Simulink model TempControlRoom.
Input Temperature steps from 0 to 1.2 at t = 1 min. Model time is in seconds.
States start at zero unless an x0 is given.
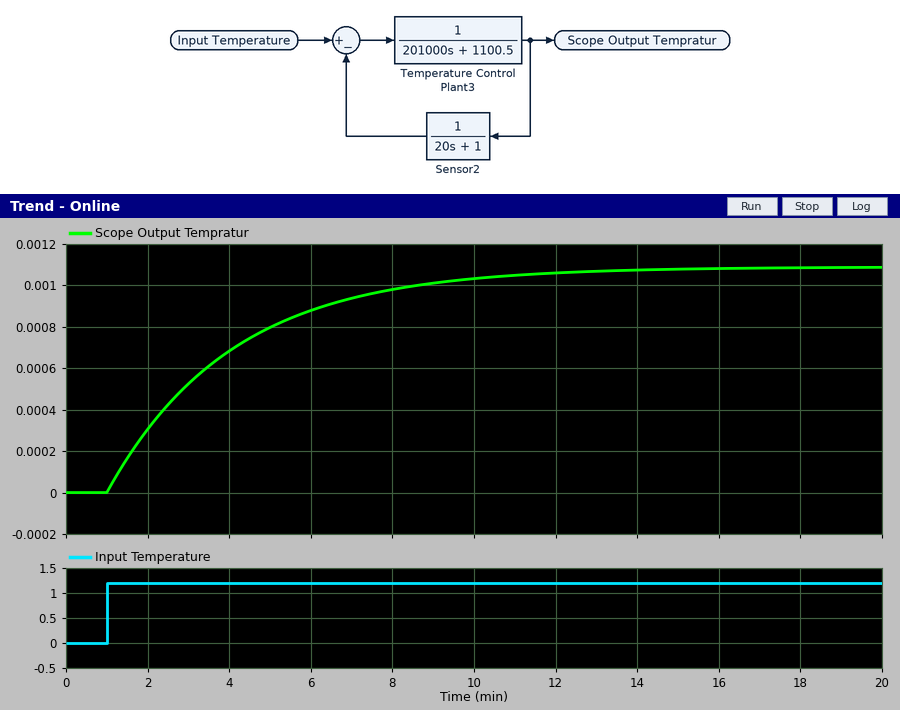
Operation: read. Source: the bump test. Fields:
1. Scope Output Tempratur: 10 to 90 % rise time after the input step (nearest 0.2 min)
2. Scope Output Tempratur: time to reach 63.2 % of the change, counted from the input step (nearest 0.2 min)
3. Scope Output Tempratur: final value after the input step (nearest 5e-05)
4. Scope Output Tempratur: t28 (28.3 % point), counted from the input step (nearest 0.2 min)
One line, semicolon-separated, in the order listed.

6.6 min; 3.0 min; 0.00110; 1.0 min
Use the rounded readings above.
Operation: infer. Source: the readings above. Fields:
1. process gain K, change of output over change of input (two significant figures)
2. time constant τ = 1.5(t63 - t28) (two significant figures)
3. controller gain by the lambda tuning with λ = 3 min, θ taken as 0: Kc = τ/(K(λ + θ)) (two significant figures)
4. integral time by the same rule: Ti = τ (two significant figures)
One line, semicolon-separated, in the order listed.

0.00092; 3.0 min; 1100; 3.0 min
